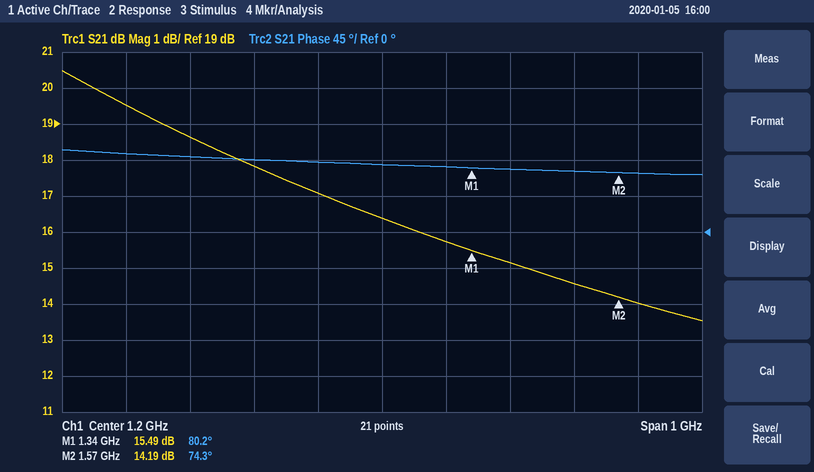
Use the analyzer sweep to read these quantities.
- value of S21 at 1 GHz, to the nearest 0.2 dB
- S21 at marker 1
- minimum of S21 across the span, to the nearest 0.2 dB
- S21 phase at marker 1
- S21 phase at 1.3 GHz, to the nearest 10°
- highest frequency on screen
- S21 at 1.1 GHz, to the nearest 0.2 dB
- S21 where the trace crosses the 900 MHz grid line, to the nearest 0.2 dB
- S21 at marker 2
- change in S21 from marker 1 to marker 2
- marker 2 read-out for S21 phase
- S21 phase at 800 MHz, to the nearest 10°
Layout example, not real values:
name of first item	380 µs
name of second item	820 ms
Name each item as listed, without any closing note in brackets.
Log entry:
value of S21 at 1 GHz, to the nearest 0.2 dB	17.8 dB
S21 at marker 1	15.49 dB
minimum of S21 across the span, to the nearest 0.2 dB	13.6 dB
S21 phase at marker 1	80.2°
S21 phase at 1.3 GHz, to the nearest 10°	80°
highest frequency on screen	1.7 GHz
S21 at 1.1 GHz, to the nearest 0.2 dB	17.0 dB
S21 where the trace crosses the 900 MHz grid line, to the nearest 0.2 dB	18.6 dB
S21 at marker 2	14.19 dB
change in S21 from marker 1 to marker 2	-1.30 dB
marker 2 read-out for S21 phase	74.3°
S21 phase at 800 MHz, to the nearest 10°	100°
